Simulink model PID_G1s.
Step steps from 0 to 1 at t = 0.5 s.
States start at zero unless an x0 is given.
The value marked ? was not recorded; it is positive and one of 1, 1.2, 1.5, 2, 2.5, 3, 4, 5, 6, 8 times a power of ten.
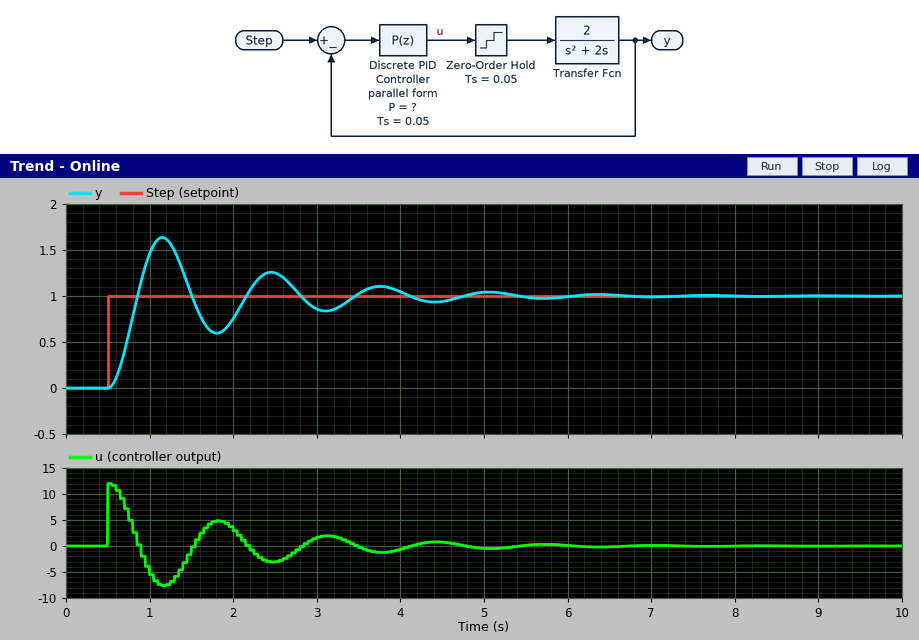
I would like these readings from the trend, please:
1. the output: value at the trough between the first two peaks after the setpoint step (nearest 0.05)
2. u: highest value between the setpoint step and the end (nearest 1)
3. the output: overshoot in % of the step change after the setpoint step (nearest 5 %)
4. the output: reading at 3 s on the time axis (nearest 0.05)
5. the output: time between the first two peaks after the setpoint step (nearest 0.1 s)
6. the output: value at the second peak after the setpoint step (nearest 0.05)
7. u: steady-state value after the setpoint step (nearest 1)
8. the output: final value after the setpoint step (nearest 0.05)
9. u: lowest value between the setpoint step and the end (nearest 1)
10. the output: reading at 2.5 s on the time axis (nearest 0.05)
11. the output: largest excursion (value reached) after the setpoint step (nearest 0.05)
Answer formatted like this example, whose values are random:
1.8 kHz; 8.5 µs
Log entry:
0.60; 12; 65 %; 0.85; 1.3 s; 1.25; 0; 1.00; -8; 1.25; 1.65
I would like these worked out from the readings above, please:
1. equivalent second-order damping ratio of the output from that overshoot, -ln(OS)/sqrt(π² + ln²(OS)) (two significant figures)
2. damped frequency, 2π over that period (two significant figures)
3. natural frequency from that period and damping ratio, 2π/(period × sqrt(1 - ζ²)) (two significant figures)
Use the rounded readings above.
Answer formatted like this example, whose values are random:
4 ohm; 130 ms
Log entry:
0.14; 4.8 rad/s; 4.9 rad/s
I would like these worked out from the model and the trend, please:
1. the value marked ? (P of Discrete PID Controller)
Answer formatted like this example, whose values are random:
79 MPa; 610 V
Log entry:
12
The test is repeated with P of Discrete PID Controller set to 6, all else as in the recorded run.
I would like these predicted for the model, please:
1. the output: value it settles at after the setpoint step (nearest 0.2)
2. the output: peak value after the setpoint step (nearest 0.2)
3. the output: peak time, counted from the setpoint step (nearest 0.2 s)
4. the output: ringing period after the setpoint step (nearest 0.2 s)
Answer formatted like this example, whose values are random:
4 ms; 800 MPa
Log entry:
1.0; 1.4; 1.0 s; 1.8 s
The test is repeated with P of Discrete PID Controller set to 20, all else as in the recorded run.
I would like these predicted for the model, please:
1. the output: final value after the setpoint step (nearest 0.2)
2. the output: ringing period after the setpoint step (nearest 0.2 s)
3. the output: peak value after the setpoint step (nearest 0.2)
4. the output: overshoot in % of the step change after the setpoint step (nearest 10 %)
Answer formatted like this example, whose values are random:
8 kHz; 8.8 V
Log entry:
1.0; 1.0 s; 1.8; 80 %
